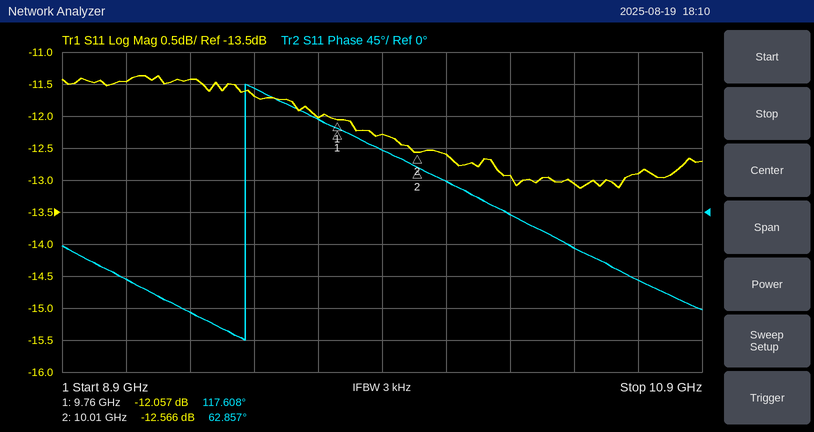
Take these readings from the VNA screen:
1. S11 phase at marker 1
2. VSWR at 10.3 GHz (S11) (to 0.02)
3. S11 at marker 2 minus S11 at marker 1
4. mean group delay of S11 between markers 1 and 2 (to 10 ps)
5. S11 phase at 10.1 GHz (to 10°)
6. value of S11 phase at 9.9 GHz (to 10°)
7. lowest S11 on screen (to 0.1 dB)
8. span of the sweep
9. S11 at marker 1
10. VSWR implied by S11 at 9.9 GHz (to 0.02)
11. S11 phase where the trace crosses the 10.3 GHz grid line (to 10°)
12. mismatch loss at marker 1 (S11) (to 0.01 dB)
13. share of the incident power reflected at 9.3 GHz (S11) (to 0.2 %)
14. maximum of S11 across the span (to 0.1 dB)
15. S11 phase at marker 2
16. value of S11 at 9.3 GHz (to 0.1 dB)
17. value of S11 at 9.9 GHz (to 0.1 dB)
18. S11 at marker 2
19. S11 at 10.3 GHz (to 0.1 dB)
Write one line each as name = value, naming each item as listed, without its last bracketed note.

S11 phase at marker 1 = 117.608°
VSWR at 10.3 GHz (S11) = 1.58
S11 at marker 2 minus S11 at marker 1 = -0.509 dB
mean group delay of S11 between markers 1 and 2 = 610 ps
S11 phase at 10.1 GHz = 40°
value of S11 phase at 9.9 GHz = 90°
lowest S11 on screen = -13.1 dB
span of the sweep = 2 GHz
S11 at marker 1 = -12.057 dB
VSWR implied by S11 at 9.9 GHz = 1.64
S11 phase where the trace crosses the 10.3 GHz grid line = 0°
mismatch loss at marker 1 (S11) = 0.28 dB
share of the incident power reflected at 9.3 GHz (S11) = 7.2 %
maximum of S11 across the span = -11.4 dB
S11 phase at marker 2 = 62.857°
value of S11 at 9.3 GHz = -11.4 dB
value of S11 at 9.9 GHz = -12.3 dB
S11 at marker 2 = -12.566 dB
S11 at 10.3 GHz = -12.9 dB
